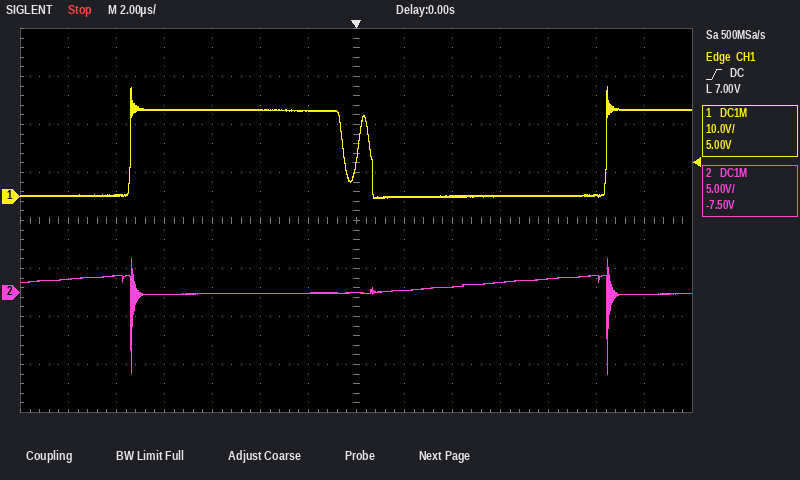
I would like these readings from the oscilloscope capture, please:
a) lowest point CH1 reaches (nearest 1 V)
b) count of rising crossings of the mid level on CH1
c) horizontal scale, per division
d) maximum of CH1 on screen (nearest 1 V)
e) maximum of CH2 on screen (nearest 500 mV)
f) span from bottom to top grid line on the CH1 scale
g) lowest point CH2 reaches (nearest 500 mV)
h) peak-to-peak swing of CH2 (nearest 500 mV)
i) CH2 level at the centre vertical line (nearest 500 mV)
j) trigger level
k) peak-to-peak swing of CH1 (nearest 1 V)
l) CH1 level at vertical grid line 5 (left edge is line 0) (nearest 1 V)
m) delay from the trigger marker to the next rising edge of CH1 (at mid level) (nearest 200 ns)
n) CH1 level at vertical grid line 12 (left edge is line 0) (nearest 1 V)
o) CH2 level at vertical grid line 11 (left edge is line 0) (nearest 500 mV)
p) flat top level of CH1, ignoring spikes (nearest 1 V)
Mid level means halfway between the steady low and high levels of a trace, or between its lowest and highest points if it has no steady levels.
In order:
0 V
3
2 µs
23 V
3.5 V
80 V
-8.5 V
12.0 V
0.0 V
7.00 V
23 V
18 V
10.4 µs
0 V
1.5 V
18 V
